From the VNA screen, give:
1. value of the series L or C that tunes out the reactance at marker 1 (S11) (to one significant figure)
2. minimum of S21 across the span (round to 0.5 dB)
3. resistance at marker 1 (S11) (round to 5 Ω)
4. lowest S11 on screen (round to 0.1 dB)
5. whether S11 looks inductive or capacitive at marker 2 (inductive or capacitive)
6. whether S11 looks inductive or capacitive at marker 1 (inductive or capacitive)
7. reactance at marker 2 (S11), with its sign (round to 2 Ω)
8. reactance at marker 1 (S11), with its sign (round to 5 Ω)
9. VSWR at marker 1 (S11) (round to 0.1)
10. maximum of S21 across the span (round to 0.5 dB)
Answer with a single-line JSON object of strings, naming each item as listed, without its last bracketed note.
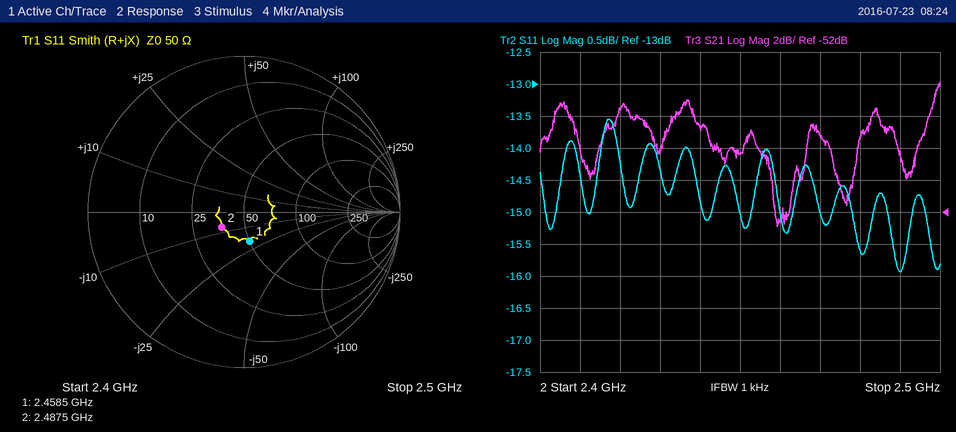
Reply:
{"value of the series L or C that tunes out the reactance at marker 1 (S11)": "1 nH", "minimum of S21 across the span": "-53.0 dB", "resistance at marker 1 (S11)": "50 Ω", "lowest S11 on screen": "-15.9 dB", "whether S11 looks inductive or capacitive at marker 2": "capacitive", "whether S11 looks inductive or capacitive at marker 1": "capacitive", "reactance at marker 2 (S11), with its sign": "-8 Ω", "reactance at marker 1 (S11), with its sign": "-20 Ω", "VSWR at marker 1 (S11)": "1.5", "maximum of S21 across the span": "-44.0 dB"}
